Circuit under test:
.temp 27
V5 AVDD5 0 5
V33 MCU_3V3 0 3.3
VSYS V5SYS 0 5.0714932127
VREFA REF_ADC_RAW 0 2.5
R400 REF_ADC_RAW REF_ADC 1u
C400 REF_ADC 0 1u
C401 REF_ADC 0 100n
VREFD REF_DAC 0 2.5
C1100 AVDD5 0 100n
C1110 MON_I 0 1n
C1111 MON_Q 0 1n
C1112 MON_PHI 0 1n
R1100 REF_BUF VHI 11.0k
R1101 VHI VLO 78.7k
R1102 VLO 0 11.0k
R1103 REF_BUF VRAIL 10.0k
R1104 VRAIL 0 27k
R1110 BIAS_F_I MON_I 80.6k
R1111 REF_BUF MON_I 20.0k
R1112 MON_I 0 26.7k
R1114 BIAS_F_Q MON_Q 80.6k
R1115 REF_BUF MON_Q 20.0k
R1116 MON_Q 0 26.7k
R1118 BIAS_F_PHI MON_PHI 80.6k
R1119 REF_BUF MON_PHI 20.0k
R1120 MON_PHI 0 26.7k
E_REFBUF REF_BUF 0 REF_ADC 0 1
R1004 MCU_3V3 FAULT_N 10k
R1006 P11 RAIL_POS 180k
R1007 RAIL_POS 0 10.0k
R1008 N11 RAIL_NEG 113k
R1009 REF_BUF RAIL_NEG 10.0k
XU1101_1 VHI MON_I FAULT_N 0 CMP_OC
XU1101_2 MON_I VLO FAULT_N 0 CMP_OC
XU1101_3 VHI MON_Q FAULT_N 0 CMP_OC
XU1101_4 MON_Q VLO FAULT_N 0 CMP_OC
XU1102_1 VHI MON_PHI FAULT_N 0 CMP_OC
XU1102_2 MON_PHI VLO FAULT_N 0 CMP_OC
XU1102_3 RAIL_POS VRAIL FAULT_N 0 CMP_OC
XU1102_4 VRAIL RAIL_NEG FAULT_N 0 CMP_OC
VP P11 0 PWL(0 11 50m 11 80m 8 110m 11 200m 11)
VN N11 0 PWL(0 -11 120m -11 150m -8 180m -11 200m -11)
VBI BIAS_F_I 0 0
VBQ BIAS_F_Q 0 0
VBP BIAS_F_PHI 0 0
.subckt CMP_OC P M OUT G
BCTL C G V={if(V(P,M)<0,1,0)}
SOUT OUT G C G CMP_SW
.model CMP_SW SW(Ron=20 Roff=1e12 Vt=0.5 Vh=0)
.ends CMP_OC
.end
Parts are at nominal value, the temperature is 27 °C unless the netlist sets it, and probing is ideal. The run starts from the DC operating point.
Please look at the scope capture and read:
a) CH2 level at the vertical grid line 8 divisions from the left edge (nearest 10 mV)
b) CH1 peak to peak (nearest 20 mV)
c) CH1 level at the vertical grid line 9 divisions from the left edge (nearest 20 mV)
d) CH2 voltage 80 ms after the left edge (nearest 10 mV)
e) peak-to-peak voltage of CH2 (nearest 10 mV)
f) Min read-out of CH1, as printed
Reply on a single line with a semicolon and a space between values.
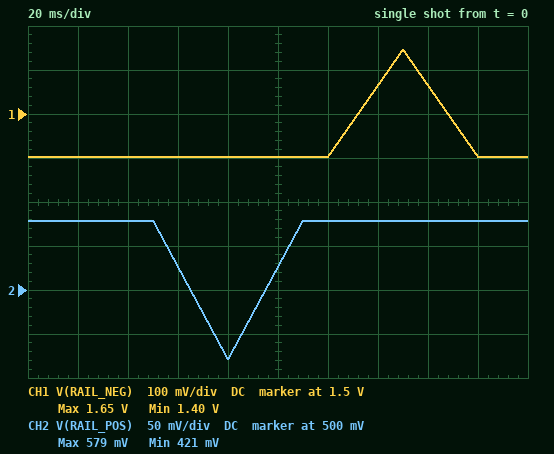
580 mV; 240 mV; 1.40 V; 420 mV; 160 mV; 1.40 V
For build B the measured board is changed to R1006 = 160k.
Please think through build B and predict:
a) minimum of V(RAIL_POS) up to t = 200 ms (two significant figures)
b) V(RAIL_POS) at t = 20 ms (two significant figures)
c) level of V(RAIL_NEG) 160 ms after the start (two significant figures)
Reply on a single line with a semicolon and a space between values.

470 mV; 650 mV; 1.6 V
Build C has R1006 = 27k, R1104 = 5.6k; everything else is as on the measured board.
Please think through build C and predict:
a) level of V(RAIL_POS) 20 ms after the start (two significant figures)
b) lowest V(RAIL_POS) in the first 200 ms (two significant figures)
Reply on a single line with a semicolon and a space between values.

3.0 V; 2.2 V
